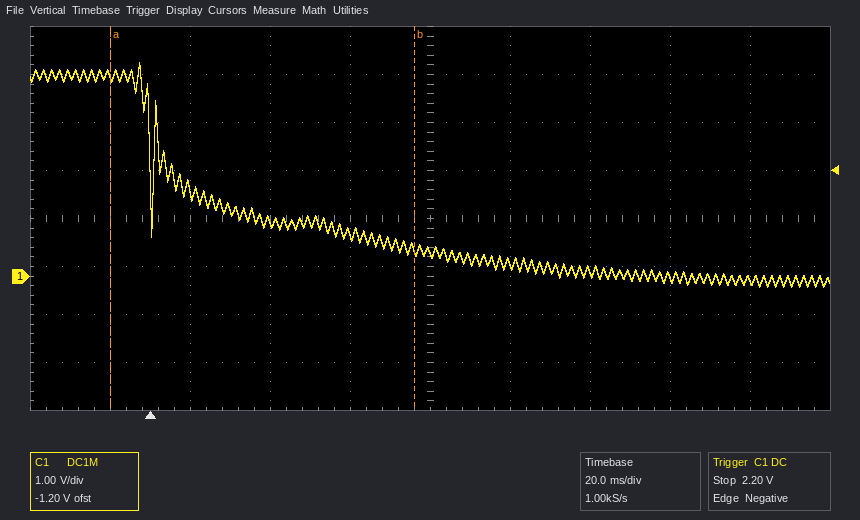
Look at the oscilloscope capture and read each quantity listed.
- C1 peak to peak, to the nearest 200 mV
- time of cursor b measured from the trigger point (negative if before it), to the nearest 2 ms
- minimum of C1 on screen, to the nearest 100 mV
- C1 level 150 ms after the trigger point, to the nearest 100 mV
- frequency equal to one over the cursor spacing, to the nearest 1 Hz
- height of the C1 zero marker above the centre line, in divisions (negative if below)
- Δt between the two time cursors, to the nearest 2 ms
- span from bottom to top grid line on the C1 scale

4.6 V
+66 ms
-200 mV
-100 mV
13 Hz
-1.2 div
76 ms
8 V
